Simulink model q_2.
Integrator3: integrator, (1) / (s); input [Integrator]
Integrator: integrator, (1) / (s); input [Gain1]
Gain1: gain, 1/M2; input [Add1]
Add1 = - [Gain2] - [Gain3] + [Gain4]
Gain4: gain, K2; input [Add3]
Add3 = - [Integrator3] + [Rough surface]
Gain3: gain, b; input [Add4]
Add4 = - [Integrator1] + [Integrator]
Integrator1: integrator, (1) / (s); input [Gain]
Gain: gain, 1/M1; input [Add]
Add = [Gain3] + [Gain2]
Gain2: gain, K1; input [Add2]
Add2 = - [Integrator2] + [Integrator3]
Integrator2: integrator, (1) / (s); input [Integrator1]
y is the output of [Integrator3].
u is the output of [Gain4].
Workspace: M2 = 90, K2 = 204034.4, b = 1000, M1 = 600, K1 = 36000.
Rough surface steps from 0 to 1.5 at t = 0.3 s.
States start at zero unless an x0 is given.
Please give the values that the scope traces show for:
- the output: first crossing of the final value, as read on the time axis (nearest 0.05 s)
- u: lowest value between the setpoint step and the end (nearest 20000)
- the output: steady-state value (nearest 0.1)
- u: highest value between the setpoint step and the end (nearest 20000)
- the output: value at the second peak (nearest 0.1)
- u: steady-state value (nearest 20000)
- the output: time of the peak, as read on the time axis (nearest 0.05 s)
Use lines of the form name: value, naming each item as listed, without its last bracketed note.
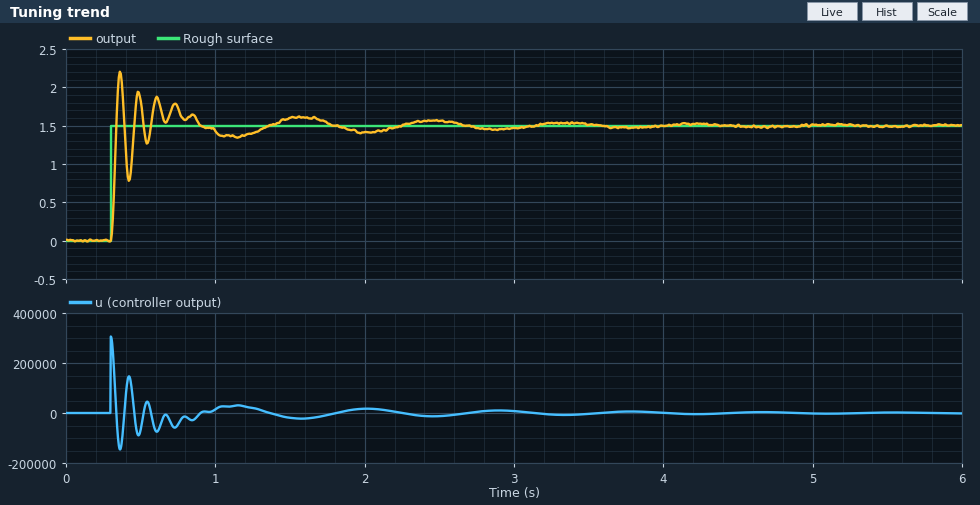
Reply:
the output: first crossing of the final value, as read on the time axis: 0.35 s
u: lowest value between the setpoint step and the end: -140000
the output: steady-state value: 1.5
u: highest value between the setpoint step and the end: 300000
the output: value at the second peak: 1.9
u: steady-state value: 0
the output: time of the peak, as read on the time axis: 0.35 s
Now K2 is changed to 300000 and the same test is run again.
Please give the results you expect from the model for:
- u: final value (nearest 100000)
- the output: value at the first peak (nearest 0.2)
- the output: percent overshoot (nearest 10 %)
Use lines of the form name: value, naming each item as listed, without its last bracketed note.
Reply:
u: final value: 0
the output: value at the first peak: 2.4
the output: percent overshoot: 60 %
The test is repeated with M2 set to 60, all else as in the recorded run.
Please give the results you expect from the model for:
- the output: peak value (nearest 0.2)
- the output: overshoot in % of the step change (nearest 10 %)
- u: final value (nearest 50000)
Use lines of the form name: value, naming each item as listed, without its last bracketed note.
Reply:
the output: peak value: 2.2
the output: overshoot in % of the step change: 40 %
u: final value: 0
